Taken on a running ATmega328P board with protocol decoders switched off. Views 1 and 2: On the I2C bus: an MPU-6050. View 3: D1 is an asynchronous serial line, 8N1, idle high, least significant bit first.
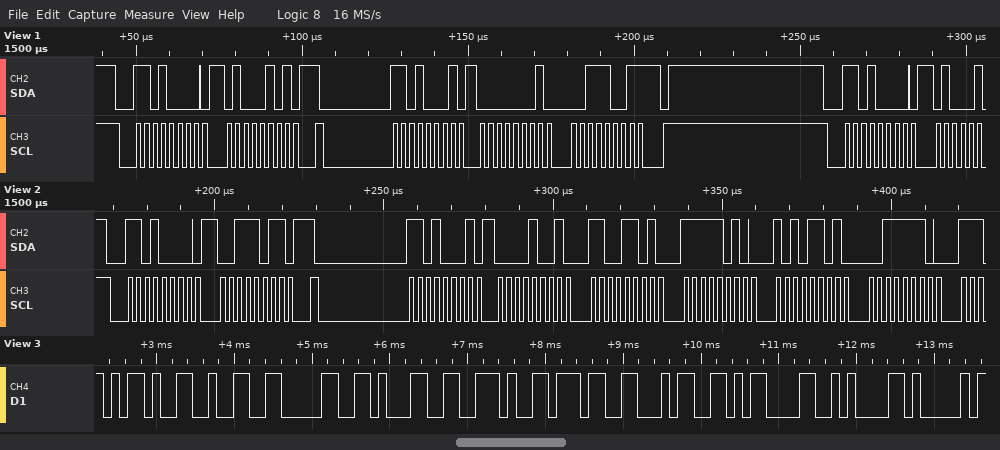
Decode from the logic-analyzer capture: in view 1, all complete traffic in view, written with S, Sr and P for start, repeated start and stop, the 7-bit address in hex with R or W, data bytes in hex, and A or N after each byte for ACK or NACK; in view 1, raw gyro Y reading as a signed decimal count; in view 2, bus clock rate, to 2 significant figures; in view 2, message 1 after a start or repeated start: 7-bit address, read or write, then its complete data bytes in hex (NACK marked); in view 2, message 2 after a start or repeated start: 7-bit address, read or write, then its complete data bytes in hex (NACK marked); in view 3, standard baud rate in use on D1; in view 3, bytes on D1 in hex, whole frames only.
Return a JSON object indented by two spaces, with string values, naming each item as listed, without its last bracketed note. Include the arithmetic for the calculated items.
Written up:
{
  "in view 1, all complete traffic in view, written with S, Sr and P for start, repeated start and stop, the 7-bit address in hex with R or W, data bytes in hex, and A or N after each byte for ACK or NACK": "S 68W A 45 A Sr 68R A 01 A 39 N P S 68W A",
  "in view 1, raw gyro Y reading as a signed decimal count": "0x0139 = 313",
  "in view 2, bus clock rate, to 2 significant figures": "400 kHz",
  "in view 2, message 1 after a start or repeated start: 7-bit address, read or write, then its complete data bytes in hex": "0x68 write: 3B",
  "in view 2, message 2 after a start or repeated start: 7-bit address, read or write, then its complete data bytes in hex": "0x68 read: 09 CD FA AD 3E",
  "in view 3, standard baud rate in use on D1": "9600 baud",
  "in view 3, bytes on D1 in hex, whole frames only": "0x2D 0x32 0x30 0x31 0x2E 0x37 0x34 0x0D 0x0A 0x41"
}
